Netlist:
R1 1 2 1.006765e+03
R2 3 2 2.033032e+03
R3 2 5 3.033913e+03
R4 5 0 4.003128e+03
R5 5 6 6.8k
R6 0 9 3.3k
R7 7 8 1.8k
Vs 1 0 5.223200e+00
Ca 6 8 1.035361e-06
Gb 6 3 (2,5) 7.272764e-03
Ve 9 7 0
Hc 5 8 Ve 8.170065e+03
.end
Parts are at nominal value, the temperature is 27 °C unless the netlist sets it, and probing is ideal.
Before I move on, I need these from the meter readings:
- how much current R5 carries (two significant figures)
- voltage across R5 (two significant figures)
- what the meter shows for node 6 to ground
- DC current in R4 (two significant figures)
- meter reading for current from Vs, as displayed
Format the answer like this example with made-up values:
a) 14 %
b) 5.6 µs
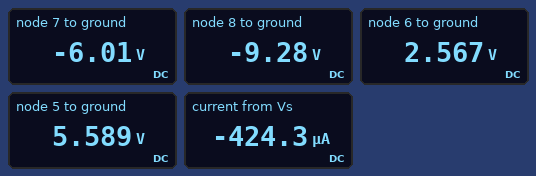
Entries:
a) 440 µA
b) 3.0 V
c) 2.567 V
d) 1.4 mA
e) -424.3 µA
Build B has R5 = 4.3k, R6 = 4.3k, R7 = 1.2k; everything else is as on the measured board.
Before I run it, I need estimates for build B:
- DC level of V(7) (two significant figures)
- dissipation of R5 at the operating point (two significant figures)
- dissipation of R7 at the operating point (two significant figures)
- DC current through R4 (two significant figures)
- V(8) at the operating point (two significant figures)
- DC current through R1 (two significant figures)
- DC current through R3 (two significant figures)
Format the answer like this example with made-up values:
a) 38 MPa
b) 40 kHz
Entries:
a) -9.4 V
b) 2.5 mW
c) 5.8 mW
d) 1.5 mA
e) -12 V
f) 730 µA
g) 35 µA
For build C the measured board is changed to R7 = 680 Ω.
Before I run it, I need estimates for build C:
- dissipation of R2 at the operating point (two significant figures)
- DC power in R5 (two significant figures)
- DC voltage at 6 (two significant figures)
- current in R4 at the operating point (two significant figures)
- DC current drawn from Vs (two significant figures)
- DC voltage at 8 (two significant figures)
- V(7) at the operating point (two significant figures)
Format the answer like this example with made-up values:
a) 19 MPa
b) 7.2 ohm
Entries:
a) 7.4 µW
b) 25 µW
c) 5.6 V
d) 1.3 mA
e) 58 µA
f) -4.9 V
g) -4.1 V
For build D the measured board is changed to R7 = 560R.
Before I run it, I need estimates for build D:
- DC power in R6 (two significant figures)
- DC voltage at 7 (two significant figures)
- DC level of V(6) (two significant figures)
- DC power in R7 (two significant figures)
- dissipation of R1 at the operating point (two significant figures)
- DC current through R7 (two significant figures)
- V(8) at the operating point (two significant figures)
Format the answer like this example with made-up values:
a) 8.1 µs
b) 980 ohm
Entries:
a) 4.7 mW
b) -3.9 V
c) 5.8 V
d) 800 µW
e) 8.4 µW
f) 1.2 mA
g) -4.6 V
